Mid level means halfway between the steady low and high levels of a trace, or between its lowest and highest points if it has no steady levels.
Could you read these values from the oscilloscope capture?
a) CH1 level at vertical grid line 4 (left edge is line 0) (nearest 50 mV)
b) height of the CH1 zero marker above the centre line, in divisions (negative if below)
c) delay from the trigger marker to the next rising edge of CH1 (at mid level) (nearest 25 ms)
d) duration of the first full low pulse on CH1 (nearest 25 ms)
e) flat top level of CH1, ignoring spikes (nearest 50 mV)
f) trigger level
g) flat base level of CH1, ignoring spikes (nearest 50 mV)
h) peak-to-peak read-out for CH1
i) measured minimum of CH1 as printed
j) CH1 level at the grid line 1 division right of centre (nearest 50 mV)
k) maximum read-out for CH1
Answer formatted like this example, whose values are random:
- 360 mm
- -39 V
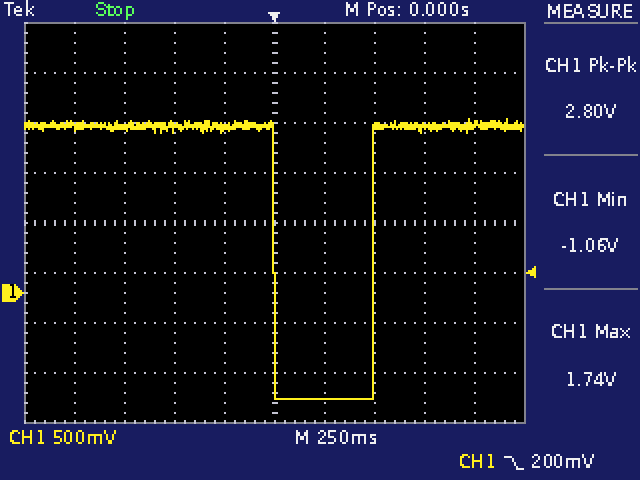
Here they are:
- 1.65 V
- -1.4 div
- 500 ms
- 500 ms
- 1.65 V
- 200 mV
- -1.05 V
- 2.80 V
- -1.06 V
- -1.05 V
- 1.74 V
